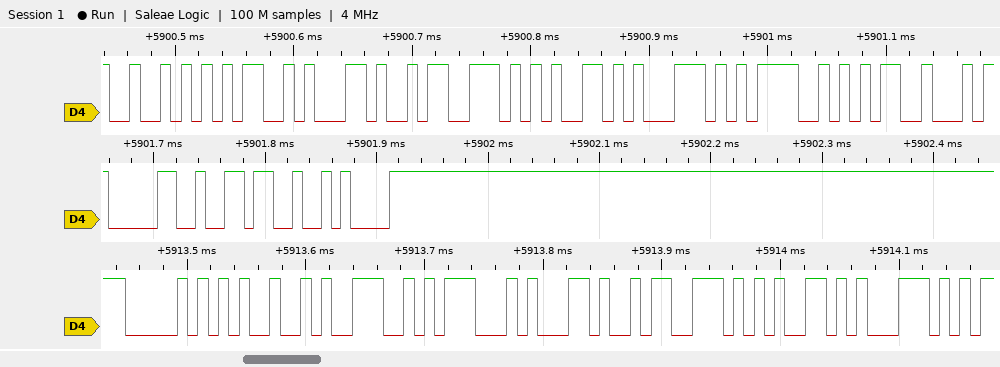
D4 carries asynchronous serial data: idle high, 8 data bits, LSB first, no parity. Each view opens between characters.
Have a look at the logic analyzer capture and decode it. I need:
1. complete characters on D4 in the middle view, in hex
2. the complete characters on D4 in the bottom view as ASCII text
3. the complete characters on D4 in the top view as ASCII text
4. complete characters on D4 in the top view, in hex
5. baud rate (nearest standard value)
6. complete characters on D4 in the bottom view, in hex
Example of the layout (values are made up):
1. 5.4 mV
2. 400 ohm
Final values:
1. 30, 36, 0A
2. "PING,seq"
3. "RM,seq=5"
4. 52, 4D, 2C, 73, 65, 71, 3D, 35
5. 115200 baud
6. 50, 49, 4E, 47, 2C, 73, 65, 71
